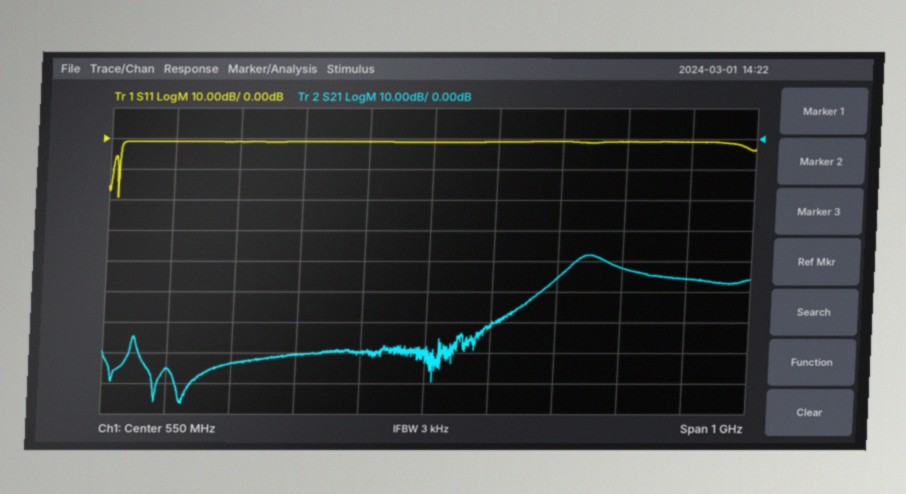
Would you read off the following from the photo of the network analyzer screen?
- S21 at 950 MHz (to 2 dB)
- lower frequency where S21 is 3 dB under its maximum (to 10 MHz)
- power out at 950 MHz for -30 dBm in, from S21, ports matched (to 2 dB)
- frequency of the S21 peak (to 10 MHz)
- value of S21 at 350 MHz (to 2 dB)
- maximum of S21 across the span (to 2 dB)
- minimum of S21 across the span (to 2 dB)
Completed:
-46 dB
770 MHz
-76 dBm
800 MHz
-70 dB
-38 dB
-86 dB
